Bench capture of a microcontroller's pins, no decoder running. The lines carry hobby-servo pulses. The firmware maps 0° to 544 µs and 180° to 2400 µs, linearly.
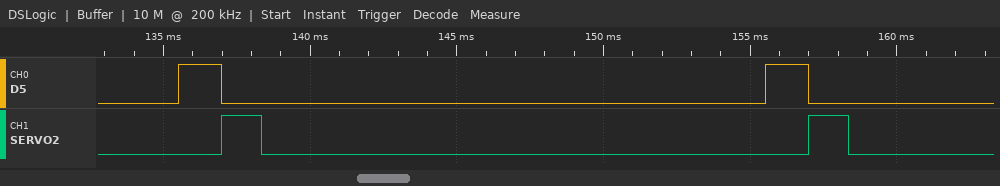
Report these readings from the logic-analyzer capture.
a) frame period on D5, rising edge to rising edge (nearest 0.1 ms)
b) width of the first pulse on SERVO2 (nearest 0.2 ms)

20.0 ms
1.4 ms
